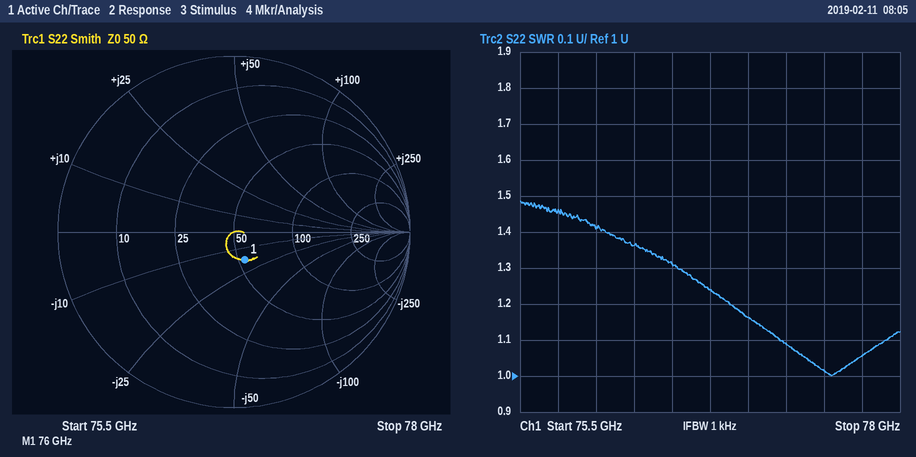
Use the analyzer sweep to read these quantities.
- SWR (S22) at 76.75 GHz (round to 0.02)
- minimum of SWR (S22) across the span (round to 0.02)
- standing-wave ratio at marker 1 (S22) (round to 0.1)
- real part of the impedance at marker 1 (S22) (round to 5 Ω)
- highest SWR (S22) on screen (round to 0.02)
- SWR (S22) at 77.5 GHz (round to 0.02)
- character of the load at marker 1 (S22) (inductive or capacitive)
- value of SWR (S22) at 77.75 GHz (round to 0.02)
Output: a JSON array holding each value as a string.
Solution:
["1.24", "1.00", "1.4", "55 Ω", "1.48", "1.02", "capacitive", "1.06"]
